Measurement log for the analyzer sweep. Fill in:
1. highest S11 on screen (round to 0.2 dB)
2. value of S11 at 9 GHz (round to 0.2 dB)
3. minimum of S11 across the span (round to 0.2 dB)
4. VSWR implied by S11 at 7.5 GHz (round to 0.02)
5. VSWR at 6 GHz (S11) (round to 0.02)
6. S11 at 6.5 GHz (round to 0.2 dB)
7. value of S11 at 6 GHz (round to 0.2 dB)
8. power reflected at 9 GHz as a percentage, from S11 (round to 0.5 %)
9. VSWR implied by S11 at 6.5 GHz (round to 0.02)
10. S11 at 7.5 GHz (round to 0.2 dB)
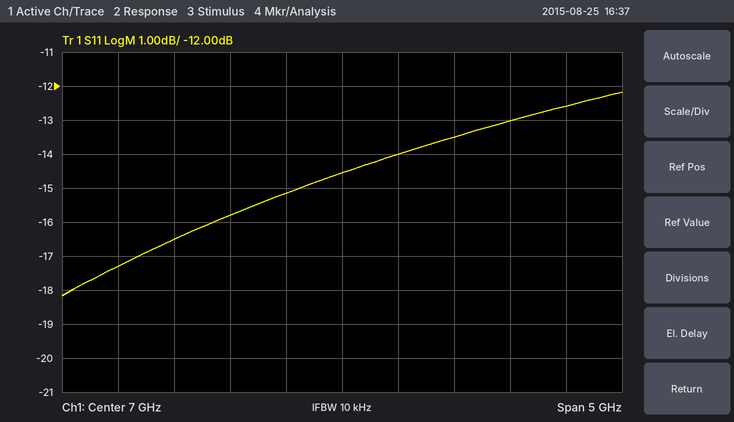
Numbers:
-12.2 dB
-12.6 dB
-18.2 dB
1.50
1.38
-15.2 dB
-15.8 dB
5.5 %
1.42
-14.0 dB
